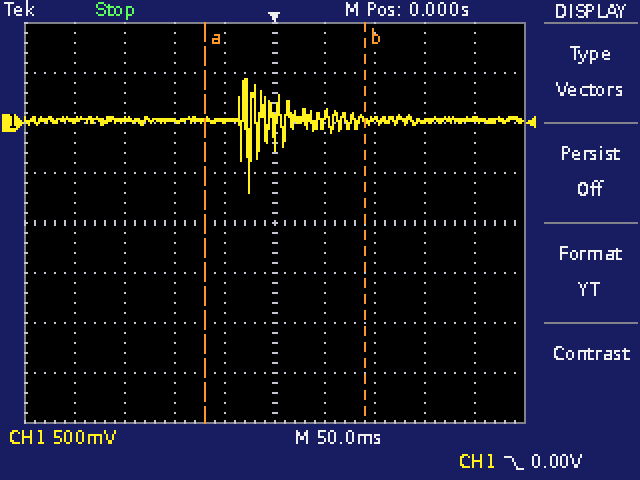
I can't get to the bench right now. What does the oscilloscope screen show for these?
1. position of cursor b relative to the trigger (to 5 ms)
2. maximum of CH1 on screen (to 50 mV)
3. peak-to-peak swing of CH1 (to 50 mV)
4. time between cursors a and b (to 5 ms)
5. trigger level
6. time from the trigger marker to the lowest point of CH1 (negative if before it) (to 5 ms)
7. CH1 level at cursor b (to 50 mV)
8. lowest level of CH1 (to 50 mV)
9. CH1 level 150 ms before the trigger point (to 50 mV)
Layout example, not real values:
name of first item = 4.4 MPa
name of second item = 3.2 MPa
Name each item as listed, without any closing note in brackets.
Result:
position of cursor b relative to the trigger = +90 ms
maximum of CH1 on screen = 450 mV
peak-to-peak swing of CH1 = 1.15 V
time between cursors a and b = 160 ms
trigger level = 0.00 V
time from the trigger marker to the lowest point of CH1 (negative if before it) = -25 ms
CH1 level at cursor b = 50 mV
lowest level of CH1 = -700 mV
CH1 level 150 ms before the trigger point = 50 mV
